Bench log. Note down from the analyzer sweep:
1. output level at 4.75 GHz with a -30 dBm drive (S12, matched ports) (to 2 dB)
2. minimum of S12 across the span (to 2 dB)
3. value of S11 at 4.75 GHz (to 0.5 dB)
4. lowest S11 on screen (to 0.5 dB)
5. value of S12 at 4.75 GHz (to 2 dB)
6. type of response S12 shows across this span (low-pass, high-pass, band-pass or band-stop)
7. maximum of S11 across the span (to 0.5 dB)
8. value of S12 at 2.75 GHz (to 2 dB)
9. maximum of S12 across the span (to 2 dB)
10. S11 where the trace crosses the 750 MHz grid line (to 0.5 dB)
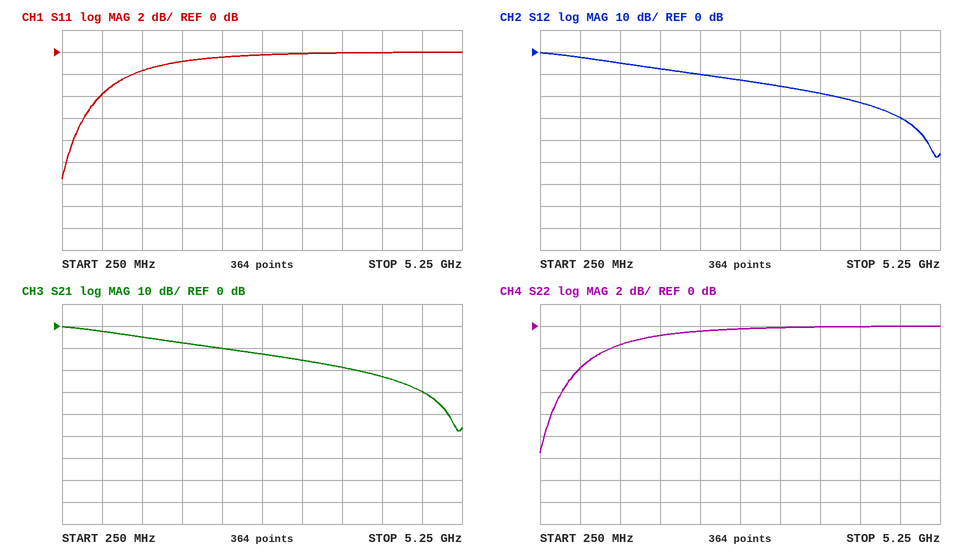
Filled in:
-60 dBm
-48 dB
0.0 dB
-11.5 dB
-30 dB
low-pass
0.0 dB
-12 dB
0 dB
-4.0 dB
